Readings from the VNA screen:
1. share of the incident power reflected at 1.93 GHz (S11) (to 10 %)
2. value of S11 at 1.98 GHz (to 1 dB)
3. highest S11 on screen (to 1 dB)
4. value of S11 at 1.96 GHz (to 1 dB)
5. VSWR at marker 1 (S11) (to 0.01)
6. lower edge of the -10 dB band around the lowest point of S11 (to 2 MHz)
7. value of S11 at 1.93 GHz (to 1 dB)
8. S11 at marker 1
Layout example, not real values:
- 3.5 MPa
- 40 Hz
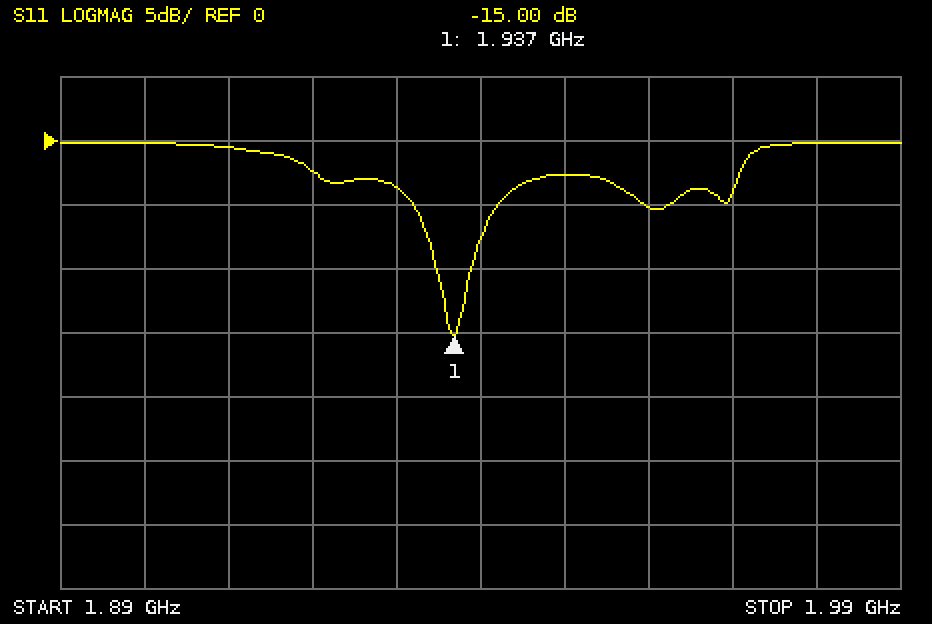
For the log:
- 40 %
- 0 dB
- 0 dB
- -5 dB
- 1.43
- 1.934 GHz
- -4 dB
- -15.00 dB
